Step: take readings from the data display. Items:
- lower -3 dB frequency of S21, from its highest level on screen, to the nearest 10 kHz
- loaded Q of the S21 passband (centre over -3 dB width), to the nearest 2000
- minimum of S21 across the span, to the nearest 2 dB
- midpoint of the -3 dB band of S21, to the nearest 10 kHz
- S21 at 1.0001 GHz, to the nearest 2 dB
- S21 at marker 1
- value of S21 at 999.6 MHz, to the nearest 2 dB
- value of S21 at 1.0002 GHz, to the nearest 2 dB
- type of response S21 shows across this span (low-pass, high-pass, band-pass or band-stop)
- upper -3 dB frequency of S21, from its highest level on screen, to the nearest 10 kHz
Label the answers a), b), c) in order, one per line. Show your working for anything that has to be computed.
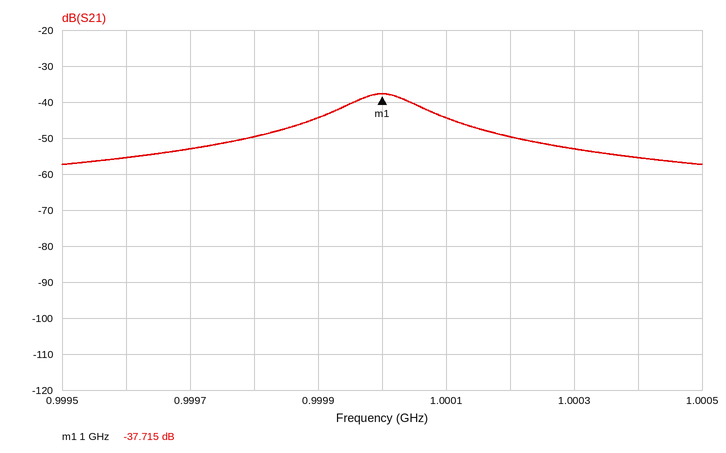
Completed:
a) 999.95 MHz
b) 1 GHz / 100 kHz ≈ 10000
c) -58 dB
d) 1.00000 GHz
e) -44 dB
f) -37.715 dB
g) -56 dB
h) -50 dB
i) band-pass
j) 1.00005 GHz
